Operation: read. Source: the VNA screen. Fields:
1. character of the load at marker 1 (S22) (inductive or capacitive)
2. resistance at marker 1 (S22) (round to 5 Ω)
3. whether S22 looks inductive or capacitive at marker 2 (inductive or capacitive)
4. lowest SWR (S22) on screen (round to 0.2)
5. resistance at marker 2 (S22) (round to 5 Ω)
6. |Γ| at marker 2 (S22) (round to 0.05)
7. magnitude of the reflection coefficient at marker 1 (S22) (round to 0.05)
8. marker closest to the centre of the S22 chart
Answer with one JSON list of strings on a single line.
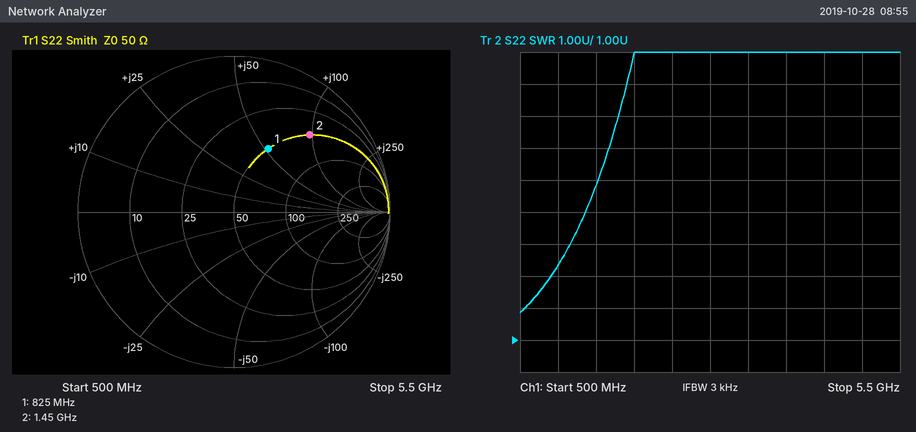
["inductive", "50 Ω", "inductive", "1.8", "50 Ω", "0.70", "0.45", "marker 1"]
